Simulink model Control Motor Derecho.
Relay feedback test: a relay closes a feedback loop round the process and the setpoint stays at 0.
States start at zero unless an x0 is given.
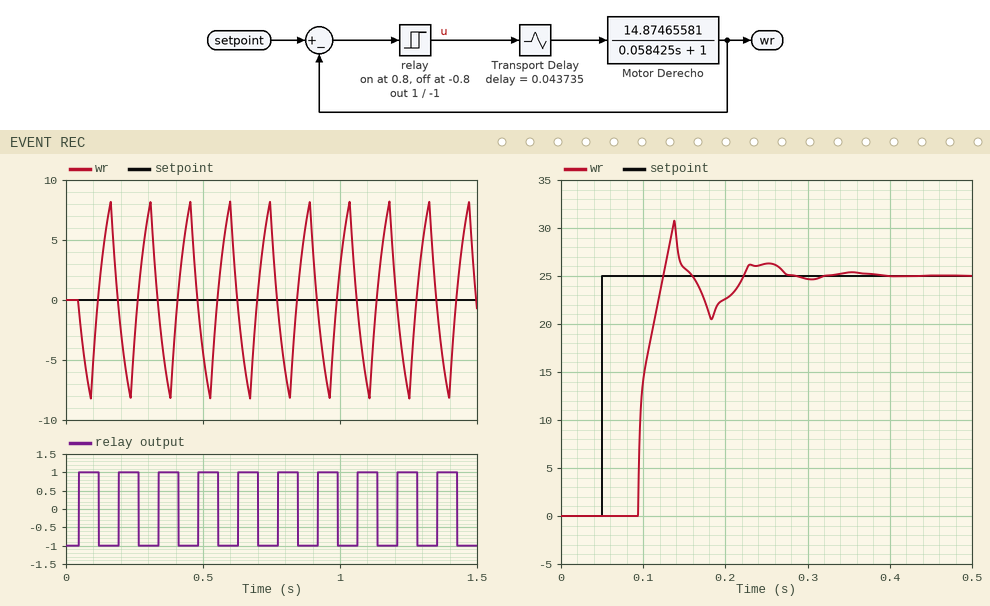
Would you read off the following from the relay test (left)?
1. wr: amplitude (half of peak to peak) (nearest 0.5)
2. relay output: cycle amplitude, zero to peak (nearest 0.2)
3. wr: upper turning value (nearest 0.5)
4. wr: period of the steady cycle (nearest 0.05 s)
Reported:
8.0
1.0
8.0
0.15 s
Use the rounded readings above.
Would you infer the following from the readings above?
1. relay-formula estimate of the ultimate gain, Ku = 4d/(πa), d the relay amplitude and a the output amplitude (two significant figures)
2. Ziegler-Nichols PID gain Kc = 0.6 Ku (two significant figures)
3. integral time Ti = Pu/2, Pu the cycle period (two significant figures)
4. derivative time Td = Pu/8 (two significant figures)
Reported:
0.16
0.096
0.075 s
0.019 s
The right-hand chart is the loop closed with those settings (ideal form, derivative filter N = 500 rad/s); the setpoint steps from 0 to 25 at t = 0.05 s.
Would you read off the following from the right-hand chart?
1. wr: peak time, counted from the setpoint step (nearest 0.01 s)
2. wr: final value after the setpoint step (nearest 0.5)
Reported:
0.09 s
25.0
